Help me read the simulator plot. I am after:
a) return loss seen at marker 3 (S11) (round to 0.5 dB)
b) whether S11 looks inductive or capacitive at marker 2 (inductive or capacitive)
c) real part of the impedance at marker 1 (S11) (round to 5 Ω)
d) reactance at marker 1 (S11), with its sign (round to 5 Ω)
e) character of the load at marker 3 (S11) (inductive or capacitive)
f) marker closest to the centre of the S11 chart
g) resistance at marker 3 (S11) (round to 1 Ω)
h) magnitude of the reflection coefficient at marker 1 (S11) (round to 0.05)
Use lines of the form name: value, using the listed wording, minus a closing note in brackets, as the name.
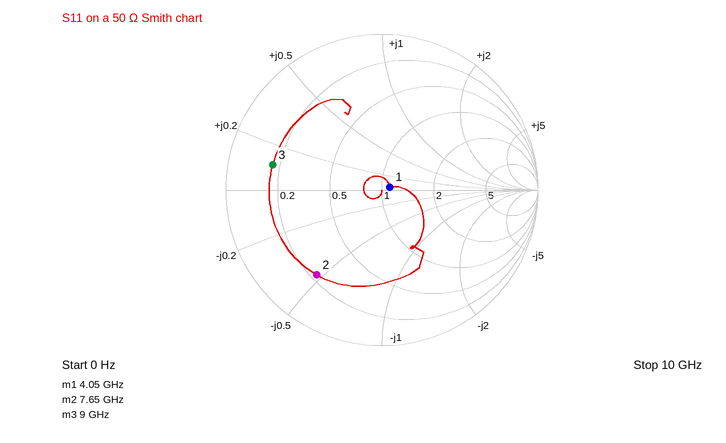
return loss seen at marker 3 (S11): 3.0 dB
whether S11 looks inductive or capacitive at marker 2: capacitive
real part of the impedance at marker 1 (S11): 55 Ω
reactance at marker 1 (S11), with its sign: 0 Ω
character of the load at marker 3 (S11): inductive
marker closest to the centre of the S11 chart: marker 1
resistance at marker 3 (S11): 8 Ω
magnitude of the reflection coefficient at marker 1 (S11): 0.05
